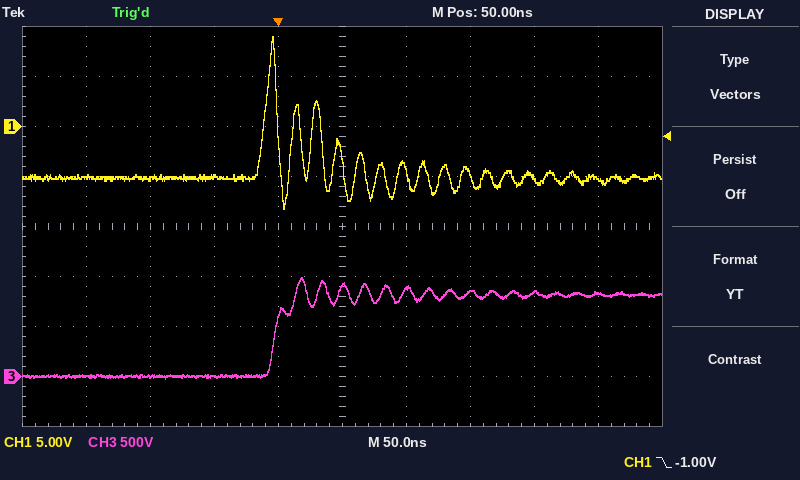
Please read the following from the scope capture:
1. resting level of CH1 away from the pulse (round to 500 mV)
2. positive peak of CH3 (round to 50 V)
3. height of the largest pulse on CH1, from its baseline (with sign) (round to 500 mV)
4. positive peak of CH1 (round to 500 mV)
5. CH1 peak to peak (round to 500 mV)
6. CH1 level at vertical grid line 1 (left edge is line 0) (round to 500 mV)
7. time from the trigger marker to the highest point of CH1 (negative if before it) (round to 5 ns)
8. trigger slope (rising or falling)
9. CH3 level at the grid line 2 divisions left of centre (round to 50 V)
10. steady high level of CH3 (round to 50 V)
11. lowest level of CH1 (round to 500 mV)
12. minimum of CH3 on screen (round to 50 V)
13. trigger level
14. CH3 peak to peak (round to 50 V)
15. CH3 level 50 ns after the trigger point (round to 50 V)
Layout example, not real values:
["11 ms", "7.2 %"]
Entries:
["-5.0 V", "1.00 kV", "+14.0 V", "9.0 V", "17.0 V", "-5.0 V", "-5 ns", "falling", "0 V", "800 V", "-8.0 V", "0 V", "-1.00 V", "1.00 kV", "900 V"]
